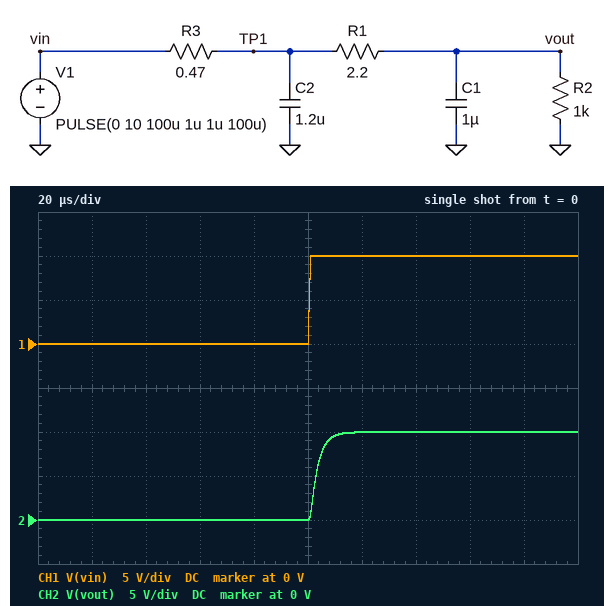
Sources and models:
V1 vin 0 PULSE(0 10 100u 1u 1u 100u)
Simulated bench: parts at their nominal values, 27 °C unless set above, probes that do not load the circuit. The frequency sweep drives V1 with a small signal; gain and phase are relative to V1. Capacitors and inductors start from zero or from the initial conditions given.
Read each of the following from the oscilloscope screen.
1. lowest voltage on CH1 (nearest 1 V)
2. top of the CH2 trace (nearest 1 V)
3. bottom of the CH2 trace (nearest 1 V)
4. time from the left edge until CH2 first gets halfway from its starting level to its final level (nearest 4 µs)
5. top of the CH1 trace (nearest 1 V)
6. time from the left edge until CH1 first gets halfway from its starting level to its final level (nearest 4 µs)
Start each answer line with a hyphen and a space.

- 0 V
- 10 V
- 0 V
- 104 µs
- 10 V
- 100 µs
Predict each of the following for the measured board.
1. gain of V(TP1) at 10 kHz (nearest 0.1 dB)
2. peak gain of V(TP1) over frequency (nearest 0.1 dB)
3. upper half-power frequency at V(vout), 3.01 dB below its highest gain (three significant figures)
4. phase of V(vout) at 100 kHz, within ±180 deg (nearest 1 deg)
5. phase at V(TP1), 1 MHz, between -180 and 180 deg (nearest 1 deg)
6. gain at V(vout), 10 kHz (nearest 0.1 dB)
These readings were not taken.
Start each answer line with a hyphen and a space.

- -0.1 dB
- 0 dB
- 55.8 kHz
- -76 deg
- -71 deg
- -0.2 dB
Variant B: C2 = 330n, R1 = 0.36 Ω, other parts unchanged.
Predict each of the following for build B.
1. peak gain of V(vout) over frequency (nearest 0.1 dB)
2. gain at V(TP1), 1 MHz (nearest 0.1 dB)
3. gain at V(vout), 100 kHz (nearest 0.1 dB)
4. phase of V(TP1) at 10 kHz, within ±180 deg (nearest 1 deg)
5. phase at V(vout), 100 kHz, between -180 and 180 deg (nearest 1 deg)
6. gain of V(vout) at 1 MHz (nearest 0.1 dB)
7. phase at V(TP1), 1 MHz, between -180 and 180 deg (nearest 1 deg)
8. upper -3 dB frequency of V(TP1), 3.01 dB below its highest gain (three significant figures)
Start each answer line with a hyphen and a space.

- 0 dB
- -8.1 dB
- -1.3 dB
- -2 deg
- -32 deg
- -16.0 dB
- -35 deg
- 205 kHz
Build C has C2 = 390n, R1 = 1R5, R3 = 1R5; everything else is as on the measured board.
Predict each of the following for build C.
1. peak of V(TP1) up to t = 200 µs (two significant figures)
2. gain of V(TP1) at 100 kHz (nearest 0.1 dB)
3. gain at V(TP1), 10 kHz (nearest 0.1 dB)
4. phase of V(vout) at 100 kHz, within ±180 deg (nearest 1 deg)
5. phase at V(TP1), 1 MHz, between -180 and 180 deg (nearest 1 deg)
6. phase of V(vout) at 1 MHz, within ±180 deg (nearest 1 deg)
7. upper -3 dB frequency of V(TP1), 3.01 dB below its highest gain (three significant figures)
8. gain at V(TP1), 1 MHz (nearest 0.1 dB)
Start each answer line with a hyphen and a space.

- 10 V
- -4.6 dB
- -0.2 dB
- -74 deg
- -62 deg
- -146 deg
- 61.7 kHz
- -12.6 dB
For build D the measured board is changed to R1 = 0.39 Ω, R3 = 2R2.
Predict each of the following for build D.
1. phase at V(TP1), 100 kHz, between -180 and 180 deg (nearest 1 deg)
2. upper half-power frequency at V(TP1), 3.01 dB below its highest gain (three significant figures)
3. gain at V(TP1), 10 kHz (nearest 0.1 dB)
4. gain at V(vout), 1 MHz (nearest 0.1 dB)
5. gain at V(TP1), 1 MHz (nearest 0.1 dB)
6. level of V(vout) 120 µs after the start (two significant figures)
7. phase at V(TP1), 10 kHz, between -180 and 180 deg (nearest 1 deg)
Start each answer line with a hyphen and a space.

- -66 deg
- 31.9 kHz
- -0.4 dB
- -34.2 dB
- -25.8 dB
- 9.8 V
- -17 deg
